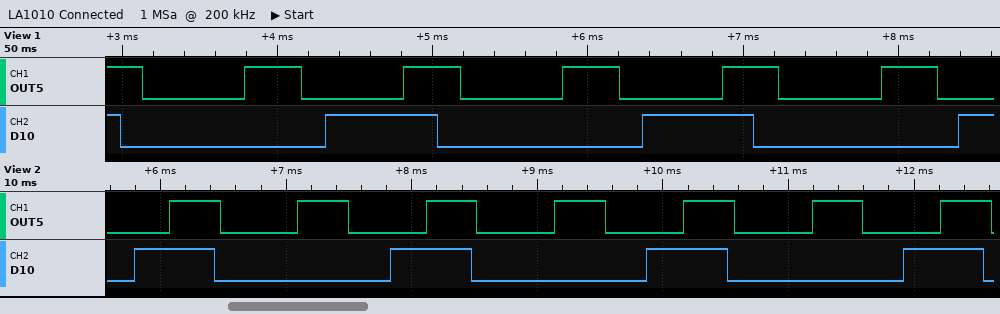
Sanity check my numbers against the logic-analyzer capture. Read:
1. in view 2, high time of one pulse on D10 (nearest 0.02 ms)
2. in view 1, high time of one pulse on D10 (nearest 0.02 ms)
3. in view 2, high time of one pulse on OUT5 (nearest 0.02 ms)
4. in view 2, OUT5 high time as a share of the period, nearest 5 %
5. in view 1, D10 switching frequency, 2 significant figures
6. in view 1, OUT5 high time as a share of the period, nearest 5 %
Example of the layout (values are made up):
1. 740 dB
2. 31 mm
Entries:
1. 0.64 ms
2. 0.72 ms
3. 0.40 ms
4. 40 %
5. 490 Hz
6. 35 %
